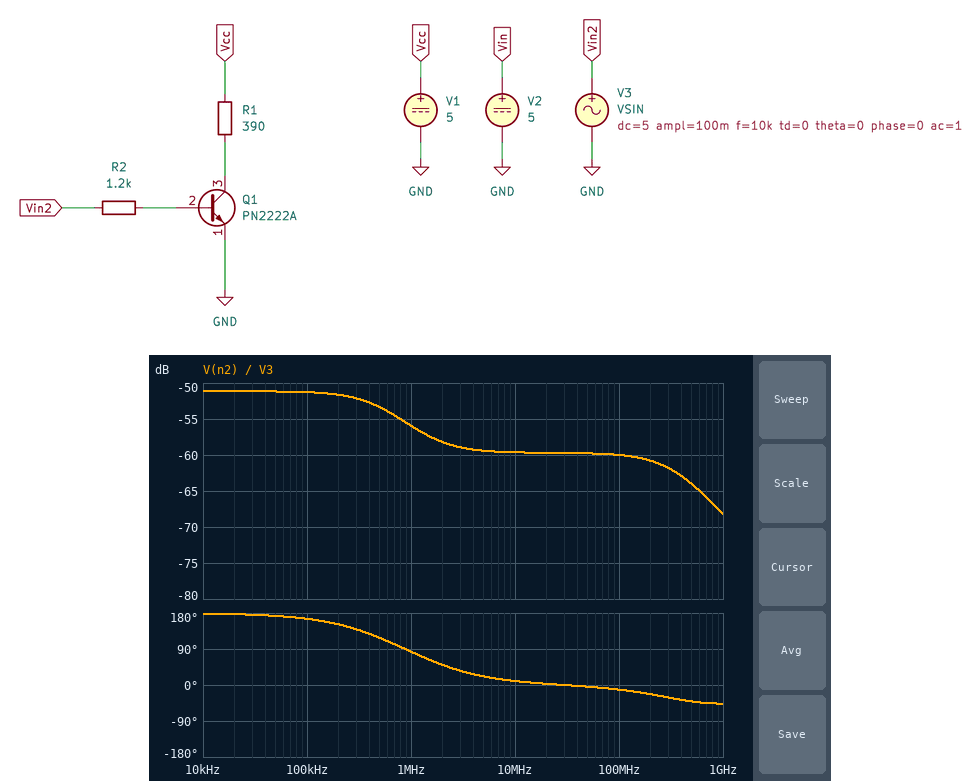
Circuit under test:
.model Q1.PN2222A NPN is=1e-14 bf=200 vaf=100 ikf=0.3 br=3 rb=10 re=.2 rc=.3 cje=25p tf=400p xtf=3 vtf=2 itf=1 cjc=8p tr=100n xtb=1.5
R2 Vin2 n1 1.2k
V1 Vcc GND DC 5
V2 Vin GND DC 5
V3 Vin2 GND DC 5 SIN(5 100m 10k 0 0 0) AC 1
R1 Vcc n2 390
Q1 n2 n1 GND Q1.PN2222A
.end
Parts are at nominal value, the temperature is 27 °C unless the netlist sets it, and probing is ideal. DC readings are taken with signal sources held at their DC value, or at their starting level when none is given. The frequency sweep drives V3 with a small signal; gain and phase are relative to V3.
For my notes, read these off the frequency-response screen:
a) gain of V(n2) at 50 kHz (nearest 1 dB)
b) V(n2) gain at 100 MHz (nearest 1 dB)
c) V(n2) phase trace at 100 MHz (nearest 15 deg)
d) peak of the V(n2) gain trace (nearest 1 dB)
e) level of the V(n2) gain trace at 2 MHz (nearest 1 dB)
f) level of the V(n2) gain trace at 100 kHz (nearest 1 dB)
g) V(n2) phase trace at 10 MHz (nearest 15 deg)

-51 dB
-60 dB
-15 deg
-51 dB
-58 dB
-51 dB
15 deg
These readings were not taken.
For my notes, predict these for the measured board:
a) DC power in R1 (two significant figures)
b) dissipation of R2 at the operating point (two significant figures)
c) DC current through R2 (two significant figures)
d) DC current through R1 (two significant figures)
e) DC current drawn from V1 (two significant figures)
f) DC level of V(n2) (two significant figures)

63 mW
15 mW
3.5 mA
13 mA
13 mA
33 mV
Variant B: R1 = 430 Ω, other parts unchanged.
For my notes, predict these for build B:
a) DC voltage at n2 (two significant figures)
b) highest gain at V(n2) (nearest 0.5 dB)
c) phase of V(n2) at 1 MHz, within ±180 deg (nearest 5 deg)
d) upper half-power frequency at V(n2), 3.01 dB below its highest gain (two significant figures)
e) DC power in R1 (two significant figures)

31 mV
-51.5 dB
80 deg
660 kHz
57 mW
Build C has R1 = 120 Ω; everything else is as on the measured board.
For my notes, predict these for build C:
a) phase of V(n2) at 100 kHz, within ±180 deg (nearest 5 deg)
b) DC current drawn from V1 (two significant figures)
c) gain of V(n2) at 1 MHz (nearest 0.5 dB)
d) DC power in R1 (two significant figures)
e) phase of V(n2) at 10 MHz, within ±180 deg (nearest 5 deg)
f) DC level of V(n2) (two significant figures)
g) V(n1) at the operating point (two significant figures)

170 deg
41 mA
-52.5 dB
200 mW
25 deg
70 mV
810 mV
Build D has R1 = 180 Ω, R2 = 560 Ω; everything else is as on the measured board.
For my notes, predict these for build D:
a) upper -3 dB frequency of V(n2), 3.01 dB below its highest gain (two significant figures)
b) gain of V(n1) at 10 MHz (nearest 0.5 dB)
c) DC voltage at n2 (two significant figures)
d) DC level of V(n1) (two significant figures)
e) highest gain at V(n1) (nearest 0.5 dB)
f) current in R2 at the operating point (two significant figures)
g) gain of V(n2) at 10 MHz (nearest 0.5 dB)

750 kHz
-34.5 dB
43 mV
840 mV
-33.5 dB
7.4 mA
-58.0 dB
